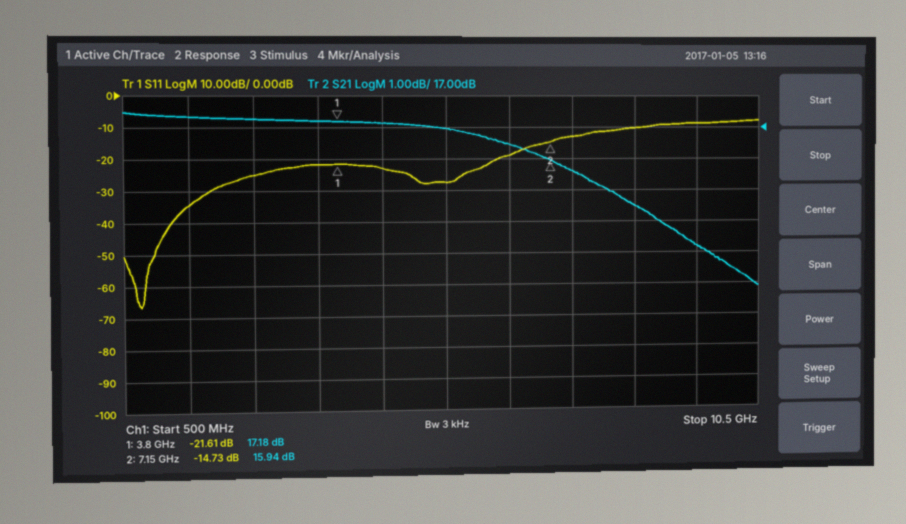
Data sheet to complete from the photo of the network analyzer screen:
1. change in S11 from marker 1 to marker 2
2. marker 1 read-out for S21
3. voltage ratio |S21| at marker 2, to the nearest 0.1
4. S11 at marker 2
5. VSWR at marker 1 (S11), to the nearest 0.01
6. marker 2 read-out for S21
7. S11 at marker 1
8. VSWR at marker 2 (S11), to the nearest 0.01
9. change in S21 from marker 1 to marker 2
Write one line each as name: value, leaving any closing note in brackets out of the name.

change in S11 from marker 1 to marker 2: 6.88 dB
marker 1 read-out for S21: 17.18 dB
voltage ratio |S21| at marker 2, to the nearest 0.1: 6.3
S11 at marker 2: -14.73 dB
VSWR at marker 1 (S11), to the nearest 0.01: 1.18
marker 2 read-out for S21: 15.94 dB
S11 at marker 1: -21.61 dB
VSWR at marker 2 (S11), to the nearest 0.01: 1.45
change in S21 from marker 1 to marker 2: -1.24 dB
